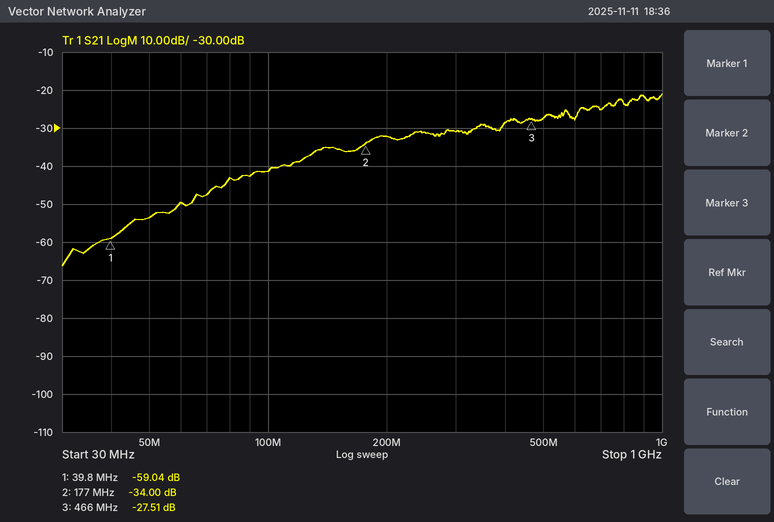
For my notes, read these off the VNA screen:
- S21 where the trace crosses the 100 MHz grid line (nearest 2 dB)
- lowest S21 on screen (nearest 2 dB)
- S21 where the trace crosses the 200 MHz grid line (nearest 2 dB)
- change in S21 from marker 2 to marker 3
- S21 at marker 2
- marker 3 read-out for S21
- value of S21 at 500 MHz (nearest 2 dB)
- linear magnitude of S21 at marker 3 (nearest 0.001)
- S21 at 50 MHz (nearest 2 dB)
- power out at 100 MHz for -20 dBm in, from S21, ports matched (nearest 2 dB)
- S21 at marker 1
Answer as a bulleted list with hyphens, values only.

- -42 dB
- -66 dB
- -32 dB
- 6.49 dB
- -34.00 dB
- -27.51 dB
- -28 dB
- 0.042
- -54 dB
- -62 dBm
- -59.04 dB
